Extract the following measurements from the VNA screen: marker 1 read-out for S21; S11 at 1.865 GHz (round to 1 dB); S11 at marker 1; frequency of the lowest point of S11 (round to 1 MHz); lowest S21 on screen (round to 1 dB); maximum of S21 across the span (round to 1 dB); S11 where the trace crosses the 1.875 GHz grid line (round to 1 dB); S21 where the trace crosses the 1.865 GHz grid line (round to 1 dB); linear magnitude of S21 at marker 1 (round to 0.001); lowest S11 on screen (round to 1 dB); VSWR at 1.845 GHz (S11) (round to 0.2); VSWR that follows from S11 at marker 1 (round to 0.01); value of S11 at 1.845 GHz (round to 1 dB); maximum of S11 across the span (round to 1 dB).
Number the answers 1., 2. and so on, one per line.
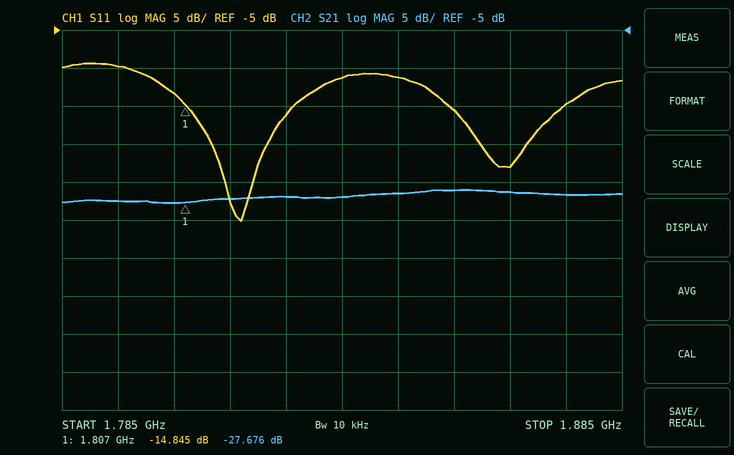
1. -27.676 dB
2. -23 dB
3. -14.845 dB
4. 1.817 GHz
5. -28 dB
6. -26 dB
7. -15 dB
8. -26 dB
9. 0.041
10. -30 dB
11. 1.8
12. 1.44
13. -11 dB
14. -9 dB
